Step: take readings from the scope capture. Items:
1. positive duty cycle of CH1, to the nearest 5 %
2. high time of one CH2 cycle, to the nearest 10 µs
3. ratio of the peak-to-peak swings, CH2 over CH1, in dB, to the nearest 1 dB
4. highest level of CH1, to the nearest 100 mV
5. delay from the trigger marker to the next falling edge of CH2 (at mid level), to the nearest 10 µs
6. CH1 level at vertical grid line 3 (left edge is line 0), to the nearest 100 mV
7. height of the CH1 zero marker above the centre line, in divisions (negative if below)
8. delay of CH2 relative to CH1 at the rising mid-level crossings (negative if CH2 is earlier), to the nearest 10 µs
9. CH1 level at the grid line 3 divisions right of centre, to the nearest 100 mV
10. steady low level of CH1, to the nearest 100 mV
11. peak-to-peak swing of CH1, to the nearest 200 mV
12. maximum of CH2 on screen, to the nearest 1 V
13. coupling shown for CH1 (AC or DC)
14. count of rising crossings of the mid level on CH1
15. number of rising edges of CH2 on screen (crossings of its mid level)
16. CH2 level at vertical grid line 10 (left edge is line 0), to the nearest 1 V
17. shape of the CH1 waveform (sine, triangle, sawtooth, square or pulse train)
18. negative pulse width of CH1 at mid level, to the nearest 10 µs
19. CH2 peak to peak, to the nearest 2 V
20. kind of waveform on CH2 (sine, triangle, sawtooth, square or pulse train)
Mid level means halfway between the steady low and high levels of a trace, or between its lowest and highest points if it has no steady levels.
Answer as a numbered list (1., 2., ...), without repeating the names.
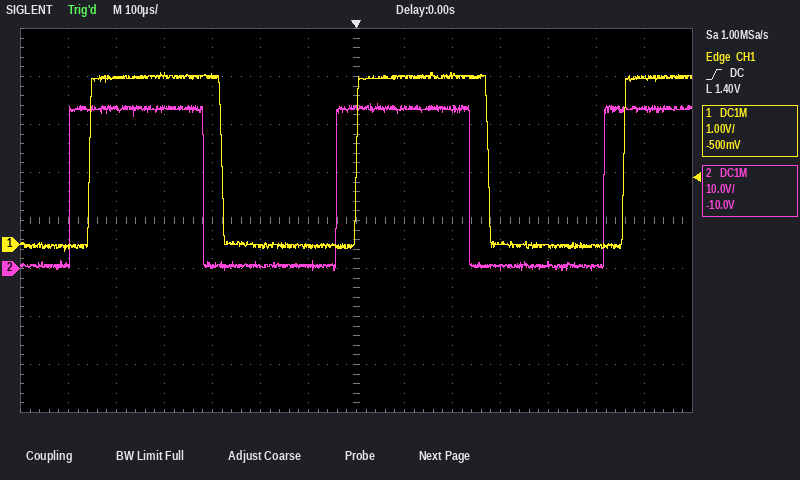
1. 50 %
2. 280 µs
3. 19 dB
4. 3.6 V
5. 240 µs
6. 3.5 V
7. -0.5 div
8. -40 µs
9. 0.0 V
10. 0.0 V
11. 3.8 V
12. 34 V
13. DC
14. 3
15. 3
16. 0 V
17. square
18. 280 µs
19. 34 V
20. square
